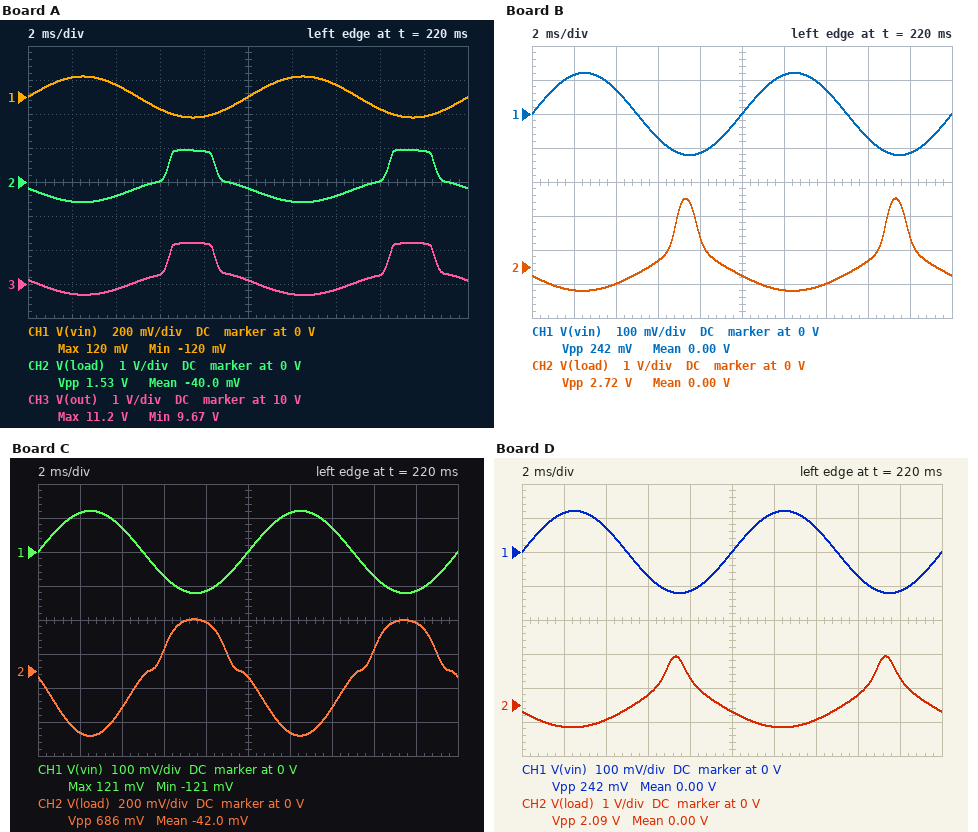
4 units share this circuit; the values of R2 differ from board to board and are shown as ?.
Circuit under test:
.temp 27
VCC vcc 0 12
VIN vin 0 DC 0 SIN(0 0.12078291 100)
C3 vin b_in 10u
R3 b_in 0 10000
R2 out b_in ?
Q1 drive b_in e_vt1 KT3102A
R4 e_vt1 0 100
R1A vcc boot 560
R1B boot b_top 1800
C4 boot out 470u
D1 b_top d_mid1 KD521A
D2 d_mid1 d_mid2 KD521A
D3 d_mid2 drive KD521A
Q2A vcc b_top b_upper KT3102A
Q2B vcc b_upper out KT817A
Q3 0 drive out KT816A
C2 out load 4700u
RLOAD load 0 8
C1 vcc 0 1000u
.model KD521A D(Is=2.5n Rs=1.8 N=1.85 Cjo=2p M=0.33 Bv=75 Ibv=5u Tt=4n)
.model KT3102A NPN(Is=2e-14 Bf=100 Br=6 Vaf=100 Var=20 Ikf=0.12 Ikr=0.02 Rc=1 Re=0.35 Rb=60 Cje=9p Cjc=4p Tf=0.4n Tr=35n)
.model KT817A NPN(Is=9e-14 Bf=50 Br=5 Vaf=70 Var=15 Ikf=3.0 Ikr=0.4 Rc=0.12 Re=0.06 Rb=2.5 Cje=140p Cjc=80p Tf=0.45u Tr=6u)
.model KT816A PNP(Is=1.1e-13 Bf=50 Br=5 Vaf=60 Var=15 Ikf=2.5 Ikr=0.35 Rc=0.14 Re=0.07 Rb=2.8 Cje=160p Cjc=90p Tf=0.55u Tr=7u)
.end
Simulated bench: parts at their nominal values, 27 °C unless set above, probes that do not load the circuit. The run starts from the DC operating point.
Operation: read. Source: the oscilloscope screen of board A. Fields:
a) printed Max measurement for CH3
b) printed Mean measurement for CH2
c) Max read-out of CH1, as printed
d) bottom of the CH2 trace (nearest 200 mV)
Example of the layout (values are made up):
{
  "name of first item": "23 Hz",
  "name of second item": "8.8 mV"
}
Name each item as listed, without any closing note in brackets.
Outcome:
{
  "printed Max measurement for CH3": "11.2 V",
  "printed Mean measurement for CH2": "-40.0 mV",
  "Max read-out of CH1, as printed": "120 mV",
  "bottom of the CH2 trace": "-600 mV"
}
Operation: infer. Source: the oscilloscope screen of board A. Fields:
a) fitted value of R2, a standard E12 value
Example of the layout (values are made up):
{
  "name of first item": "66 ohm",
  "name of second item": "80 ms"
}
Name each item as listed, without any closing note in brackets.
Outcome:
{
  "fitted value of R2, a standard E12 value": "120 kΩ"
}
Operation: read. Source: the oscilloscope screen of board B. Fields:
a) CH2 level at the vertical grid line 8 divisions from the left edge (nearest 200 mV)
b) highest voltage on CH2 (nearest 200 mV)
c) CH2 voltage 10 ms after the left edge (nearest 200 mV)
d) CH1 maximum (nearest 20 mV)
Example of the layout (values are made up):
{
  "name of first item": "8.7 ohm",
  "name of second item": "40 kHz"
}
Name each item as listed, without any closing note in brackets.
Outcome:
{
  "CH2 level at the vertical grid line 8 divisions from the left edge": "200 mV",
  "highest voltage on CH2": "2.0 V",
  "CH2 voltage 10 ms after the left edge": "-200 mV",
  "CH1 maximum": "120 mV"
}
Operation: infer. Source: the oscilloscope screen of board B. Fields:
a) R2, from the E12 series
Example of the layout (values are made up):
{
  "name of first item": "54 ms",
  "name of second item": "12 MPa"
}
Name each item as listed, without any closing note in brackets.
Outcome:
{
  "R2, from the E12 series": "33 kΩ"
}
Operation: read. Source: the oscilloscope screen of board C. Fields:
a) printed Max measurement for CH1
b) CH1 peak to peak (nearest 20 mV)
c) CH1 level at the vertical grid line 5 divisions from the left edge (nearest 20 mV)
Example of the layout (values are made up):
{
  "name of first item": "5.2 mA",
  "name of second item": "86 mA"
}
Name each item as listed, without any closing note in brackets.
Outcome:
{
  "printed Max measurement for CH1": "121 mV",
  "CH1 peak to peak": "240 mV",
  "CH1 level at the vertical grid line 5 divisions from the left edge": "0 V"
}
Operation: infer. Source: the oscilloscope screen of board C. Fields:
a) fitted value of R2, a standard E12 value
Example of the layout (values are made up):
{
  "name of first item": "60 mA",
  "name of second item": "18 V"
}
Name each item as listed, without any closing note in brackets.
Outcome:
{
  "fitted value of R2, a standard E12 value": "150 kΩ"
}
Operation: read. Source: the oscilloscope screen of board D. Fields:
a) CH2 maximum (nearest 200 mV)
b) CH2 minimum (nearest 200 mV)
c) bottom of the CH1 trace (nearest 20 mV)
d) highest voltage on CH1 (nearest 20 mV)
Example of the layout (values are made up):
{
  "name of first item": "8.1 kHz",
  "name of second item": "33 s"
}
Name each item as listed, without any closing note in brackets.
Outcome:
{
  "CH2 maximum": "1.4 V",
  "CH2 minimum": "-600 mV",
  "bottom of the CH1 trace": "-120 mV",
  "highest voltage on CH1": "120 mV"
}
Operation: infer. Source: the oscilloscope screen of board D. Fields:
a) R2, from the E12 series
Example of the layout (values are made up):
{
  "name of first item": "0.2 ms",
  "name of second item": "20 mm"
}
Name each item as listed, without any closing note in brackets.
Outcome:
{
  "R2, from the E12 series": "22 kΩ"
}
